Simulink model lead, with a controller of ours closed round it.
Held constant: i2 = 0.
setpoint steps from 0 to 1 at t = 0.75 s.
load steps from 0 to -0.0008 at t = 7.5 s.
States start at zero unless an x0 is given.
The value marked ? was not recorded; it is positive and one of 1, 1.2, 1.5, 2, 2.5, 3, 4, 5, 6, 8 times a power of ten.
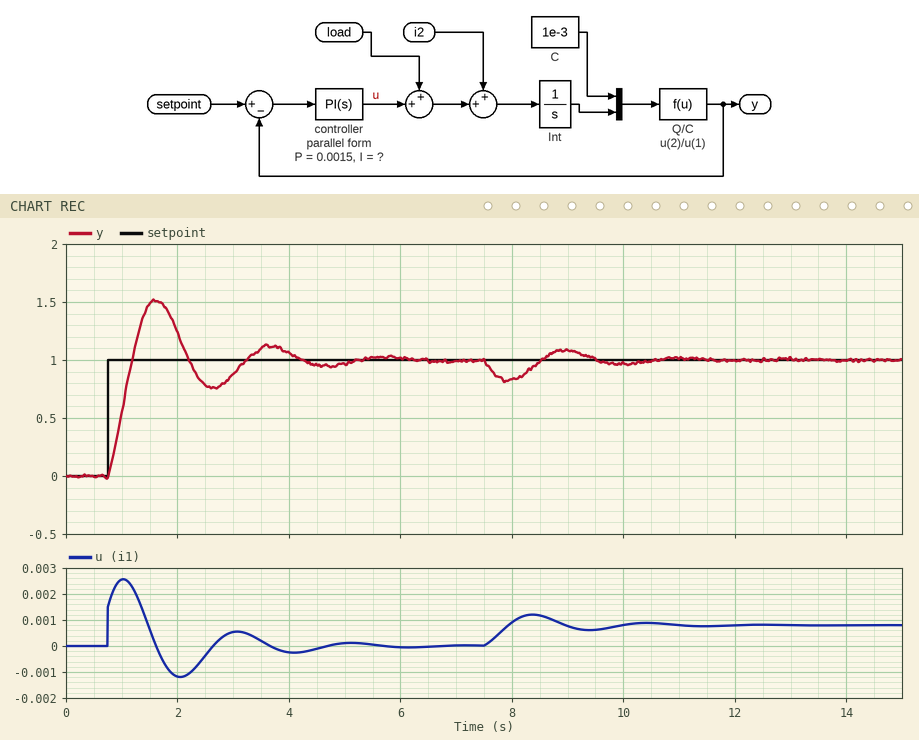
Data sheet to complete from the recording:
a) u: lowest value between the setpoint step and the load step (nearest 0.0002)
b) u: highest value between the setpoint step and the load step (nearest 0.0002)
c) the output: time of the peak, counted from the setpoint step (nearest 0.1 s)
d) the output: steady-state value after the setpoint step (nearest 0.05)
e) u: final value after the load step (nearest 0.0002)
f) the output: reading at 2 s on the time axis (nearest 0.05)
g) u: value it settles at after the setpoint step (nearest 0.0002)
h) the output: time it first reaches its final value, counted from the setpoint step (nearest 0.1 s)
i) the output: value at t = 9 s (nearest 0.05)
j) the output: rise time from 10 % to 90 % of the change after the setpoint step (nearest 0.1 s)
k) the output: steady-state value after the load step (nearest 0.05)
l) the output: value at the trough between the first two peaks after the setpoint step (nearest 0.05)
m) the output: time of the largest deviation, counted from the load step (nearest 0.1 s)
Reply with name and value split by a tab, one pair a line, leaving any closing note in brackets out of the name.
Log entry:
u: lowest value between the setpoint step and the load step	-0.0012
u: highest value between the setpoint step and the load step	0.0026
the output: time of the peak, counted from the setpoint step	0.9 s
the output: steady-state value after the setpoint step	1.00
u: final value after the load step	0.0008
the output: reading at 2 s on the time axis	1.25
u: value it settles at after the setpoint step	0.0000
the output: time it first reaches its final value, counted from the setpoint step	0.4 s
the output: value at t = 9 s	1.10
the output: rise time from 10 % to 90 % of the change after the setpoint step	0.3 s
the output: steady-state value after the load step	1.00
the output: value at the trough between the first two peaks after the setpoint step	0.75
the output: time of the largest deviation, counted from the load step	0.4 s
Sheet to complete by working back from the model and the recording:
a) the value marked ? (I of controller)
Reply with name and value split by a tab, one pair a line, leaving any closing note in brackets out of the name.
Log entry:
the value marked ?	0.01
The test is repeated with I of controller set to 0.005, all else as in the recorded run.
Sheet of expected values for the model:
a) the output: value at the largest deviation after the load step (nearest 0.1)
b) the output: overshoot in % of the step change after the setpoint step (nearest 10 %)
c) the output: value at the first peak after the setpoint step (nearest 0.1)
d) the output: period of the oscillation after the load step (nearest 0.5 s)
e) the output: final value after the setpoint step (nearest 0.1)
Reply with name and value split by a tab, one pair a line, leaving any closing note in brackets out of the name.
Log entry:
the output: value at the largest deviation after the load step	0.8
the output: overshoot in % of the step change after the setpoint step	40 %
the output: value at the first peak after the setpoint step	1.4
the output: period of the oscillation after the load step	3.0 s
the output: final value after the setpoint step	1.0
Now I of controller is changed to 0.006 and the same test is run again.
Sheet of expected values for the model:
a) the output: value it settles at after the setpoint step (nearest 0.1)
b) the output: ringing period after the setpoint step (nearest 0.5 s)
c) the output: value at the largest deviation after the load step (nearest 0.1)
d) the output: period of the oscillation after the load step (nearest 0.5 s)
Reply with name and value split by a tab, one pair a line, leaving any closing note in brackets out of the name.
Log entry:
the output: value it settles at after the setpoint step	1.0
the output: ringing period after the setpoint step	2.5 s
the output: value at the largest deviation after the load step	0.8
the output: period of the oscillation after the load step	2.5 s
